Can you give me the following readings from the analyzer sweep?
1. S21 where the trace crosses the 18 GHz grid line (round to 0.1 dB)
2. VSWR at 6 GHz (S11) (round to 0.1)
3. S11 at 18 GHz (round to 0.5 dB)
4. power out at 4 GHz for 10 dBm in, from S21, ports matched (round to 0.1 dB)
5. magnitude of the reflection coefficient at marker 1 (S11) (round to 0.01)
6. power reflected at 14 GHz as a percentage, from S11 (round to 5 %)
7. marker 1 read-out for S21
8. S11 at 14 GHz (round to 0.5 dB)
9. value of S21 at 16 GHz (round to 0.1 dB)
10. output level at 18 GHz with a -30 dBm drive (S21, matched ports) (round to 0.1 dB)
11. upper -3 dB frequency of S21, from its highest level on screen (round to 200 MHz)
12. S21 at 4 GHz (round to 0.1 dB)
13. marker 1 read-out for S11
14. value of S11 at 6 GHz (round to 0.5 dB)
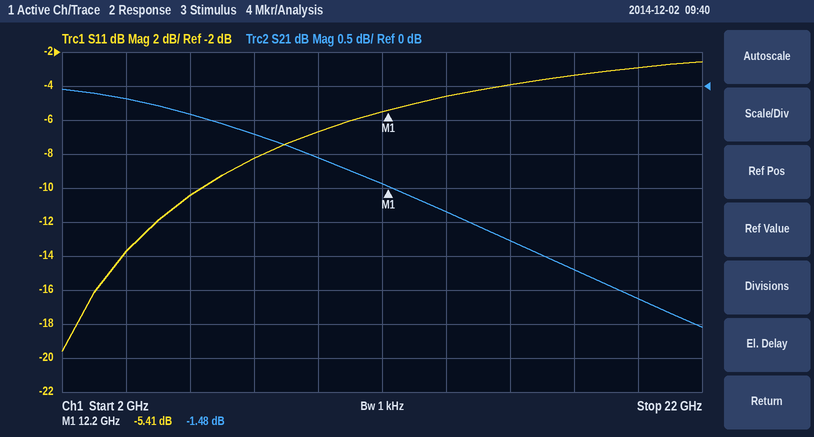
-2.7 dB
1.9
-3.5 dB
9.8 dBm
0.54
35 %
-1.48 dB
-4.5 dB
-2.3 dB
-32.7 dBm
19.6 GHz
-0.2 dB
-5.41 dB
-10.5 dB
